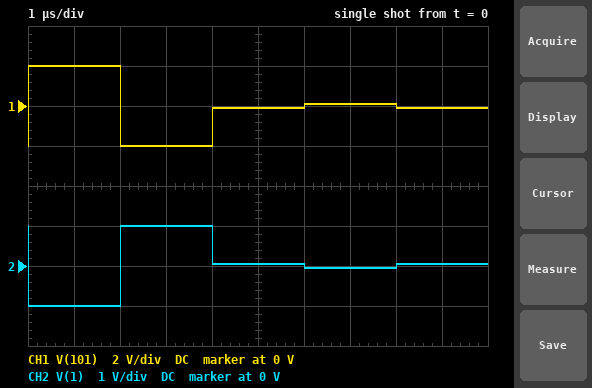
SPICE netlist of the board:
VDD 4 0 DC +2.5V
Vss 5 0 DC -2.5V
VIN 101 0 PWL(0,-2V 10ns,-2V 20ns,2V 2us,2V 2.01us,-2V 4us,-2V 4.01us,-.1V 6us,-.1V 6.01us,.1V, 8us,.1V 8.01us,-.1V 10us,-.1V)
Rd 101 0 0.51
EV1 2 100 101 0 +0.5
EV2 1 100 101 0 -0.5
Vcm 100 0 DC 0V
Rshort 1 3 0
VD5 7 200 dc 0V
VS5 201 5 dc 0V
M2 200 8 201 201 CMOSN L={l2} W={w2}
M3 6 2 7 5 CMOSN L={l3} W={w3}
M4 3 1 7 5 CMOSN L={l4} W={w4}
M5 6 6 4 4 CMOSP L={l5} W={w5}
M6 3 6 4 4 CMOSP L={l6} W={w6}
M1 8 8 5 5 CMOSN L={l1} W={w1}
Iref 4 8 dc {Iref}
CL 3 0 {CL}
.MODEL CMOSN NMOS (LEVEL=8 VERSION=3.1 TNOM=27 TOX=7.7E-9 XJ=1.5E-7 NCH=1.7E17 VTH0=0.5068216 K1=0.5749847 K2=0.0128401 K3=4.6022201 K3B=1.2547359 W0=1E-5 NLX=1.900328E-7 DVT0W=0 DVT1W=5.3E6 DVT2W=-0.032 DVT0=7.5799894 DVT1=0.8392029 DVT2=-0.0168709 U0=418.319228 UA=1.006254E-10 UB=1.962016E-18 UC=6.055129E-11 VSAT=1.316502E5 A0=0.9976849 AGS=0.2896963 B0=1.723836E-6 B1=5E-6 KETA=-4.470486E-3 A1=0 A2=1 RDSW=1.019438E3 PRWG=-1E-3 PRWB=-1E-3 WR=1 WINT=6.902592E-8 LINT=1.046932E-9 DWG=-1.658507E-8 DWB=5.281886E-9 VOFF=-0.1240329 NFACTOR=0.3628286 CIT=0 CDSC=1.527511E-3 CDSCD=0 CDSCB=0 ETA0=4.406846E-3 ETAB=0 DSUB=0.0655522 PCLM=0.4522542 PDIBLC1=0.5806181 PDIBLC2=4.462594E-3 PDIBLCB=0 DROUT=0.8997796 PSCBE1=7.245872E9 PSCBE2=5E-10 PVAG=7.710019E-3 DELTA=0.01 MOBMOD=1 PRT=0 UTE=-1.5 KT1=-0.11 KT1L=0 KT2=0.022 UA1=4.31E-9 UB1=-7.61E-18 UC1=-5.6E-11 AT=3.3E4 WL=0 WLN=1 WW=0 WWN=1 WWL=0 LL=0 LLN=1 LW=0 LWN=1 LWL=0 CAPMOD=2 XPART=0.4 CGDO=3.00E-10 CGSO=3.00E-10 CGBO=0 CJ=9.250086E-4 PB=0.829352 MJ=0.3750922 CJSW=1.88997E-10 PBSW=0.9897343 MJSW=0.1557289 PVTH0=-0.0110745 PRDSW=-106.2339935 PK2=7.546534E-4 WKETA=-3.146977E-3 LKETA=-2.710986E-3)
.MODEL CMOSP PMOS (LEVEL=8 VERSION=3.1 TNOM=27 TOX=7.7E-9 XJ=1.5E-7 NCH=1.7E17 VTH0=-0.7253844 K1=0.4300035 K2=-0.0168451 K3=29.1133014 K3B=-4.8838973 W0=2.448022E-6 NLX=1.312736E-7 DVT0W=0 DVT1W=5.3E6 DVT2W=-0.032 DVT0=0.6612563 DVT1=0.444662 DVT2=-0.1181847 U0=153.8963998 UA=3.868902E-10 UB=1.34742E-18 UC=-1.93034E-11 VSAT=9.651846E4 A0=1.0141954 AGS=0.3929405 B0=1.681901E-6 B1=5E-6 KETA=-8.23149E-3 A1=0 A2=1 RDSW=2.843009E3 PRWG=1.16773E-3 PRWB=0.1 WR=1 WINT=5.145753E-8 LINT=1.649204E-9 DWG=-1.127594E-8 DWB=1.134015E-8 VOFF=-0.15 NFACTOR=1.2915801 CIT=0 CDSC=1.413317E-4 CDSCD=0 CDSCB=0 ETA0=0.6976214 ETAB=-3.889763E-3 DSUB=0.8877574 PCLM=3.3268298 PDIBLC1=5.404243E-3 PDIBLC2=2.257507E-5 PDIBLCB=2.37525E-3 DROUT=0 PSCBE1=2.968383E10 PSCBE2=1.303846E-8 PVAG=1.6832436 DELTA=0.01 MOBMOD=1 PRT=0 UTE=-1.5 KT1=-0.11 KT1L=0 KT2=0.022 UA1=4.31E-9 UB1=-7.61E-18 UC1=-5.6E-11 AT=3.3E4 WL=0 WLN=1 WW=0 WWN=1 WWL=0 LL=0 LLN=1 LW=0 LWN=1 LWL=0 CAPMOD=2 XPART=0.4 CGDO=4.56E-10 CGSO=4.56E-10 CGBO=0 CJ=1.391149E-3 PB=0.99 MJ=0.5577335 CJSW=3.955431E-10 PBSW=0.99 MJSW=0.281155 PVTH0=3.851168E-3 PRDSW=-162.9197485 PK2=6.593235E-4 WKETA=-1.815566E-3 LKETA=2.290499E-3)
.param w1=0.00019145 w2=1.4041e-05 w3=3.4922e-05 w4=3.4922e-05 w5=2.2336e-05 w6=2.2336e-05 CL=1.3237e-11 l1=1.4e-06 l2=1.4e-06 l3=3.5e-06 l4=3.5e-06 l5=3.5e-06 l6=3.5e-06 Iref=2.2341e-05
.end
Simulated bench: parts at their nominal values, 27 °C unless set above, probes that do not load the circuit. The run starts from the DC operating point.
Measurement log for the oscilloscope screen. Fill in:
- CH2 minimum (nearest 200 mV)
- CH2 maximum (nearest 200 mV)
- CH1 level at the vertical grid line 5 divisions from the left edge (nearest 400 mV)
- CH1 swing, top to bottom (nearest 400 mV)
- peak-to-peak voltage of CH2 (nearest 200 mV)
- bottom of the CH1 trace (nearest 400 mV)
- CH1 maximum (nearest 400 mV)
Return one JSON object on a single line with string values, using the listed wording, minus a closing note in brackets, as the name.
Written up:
{"CH2 minimum": "-1.0 V", "CH2 maximum": "1.0 V", "CH1 level at the vertical grid line 5 divisions from the left edge": "0 V", "CH1 swing, top to bottom": "4.0 V", "peak-to-peak voltage of CH2": "2.0 V", "bottom of the CH1 trace": "-2.0 V", "CH1 maximum": "2.0 V"}
